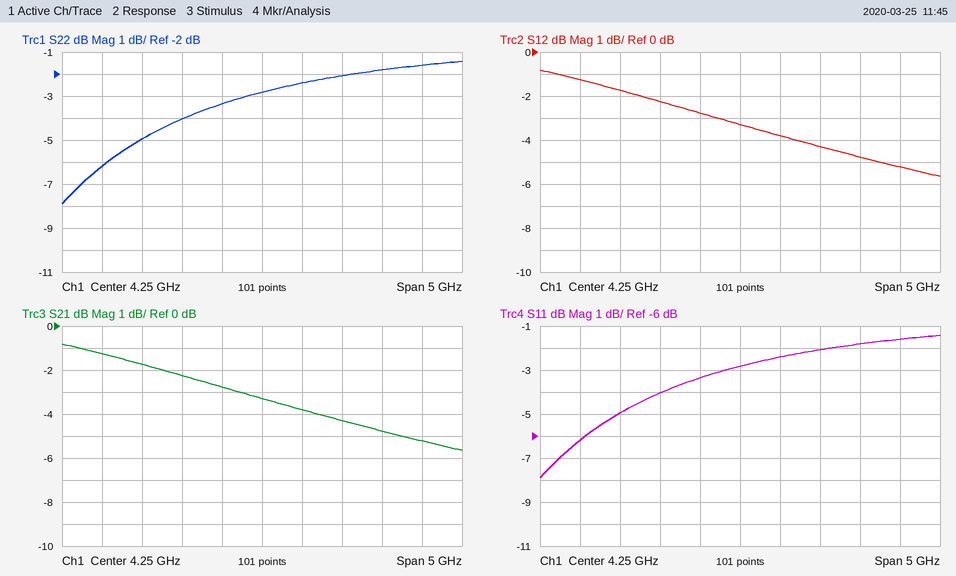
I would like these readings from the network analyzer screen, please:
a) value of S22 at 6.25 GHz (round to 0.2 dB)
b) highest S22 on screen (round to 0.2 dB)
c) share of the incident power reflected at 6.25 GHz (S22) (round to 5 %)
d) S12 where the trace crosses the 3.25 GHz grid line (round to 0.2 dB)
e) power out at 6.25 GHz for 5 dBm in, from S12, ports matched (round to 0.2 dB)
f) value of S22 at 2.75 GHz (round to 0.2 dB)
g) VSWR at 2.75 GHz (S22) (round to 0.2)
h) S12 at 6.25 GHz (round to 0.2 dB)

-1.6 dB
-1.4 dB
70 %
-2.2 dB
-0.2 dBm
-5.0 dB
3.6
-5.2 dB
